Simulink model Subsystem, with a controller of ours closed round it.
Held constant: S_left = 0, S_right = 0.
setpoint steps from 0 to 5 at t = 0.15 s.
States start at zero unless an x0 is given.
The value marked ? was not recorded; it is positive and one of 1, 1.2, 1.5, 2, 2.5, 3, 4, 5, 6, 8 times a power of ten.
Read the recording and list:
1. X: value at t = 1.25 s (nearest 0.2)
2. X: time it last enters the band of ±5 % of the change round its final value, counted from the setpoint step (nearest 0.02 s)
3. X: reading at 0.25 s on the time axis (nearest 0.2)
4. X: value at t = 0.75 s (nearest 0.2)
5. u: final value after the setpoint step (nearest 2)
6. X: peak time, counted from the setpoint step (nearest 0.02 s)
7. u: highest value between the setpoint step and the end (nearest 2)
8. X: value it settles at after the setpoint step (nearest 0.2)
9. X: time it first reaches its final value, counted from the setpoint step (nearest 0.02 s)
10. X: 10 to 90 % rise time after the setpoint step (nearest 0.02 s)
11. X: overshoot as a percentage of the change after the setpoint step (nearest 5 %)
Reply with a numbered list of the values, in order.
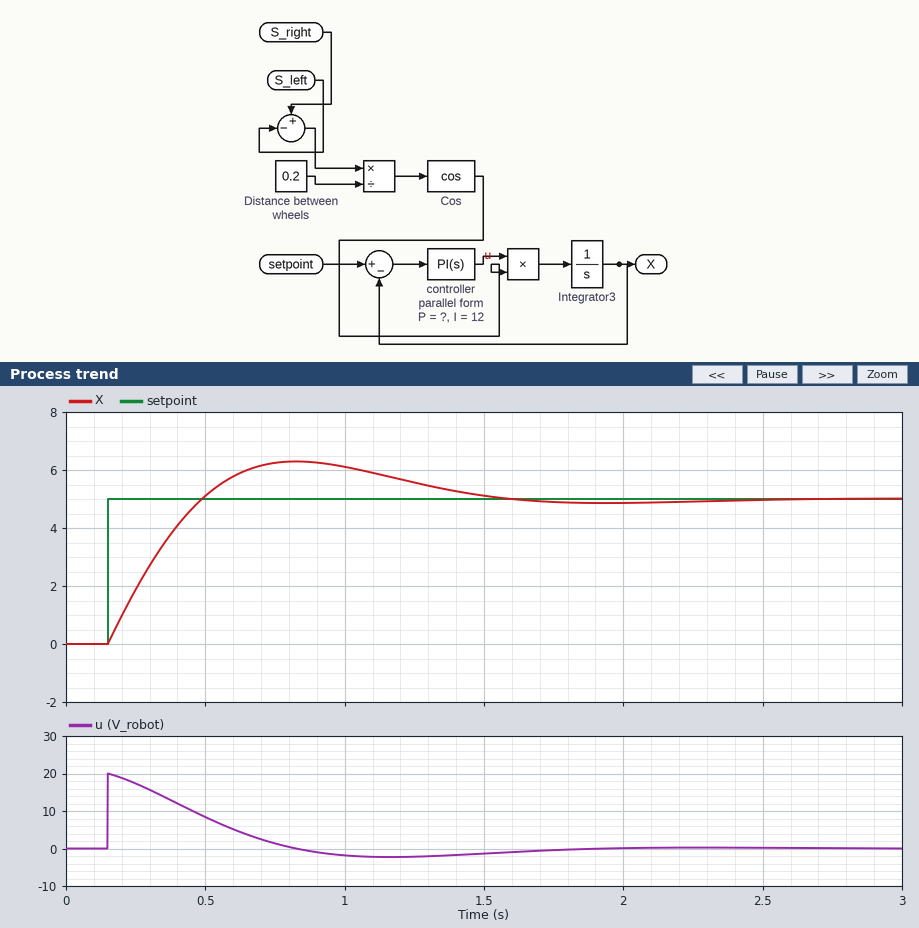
1. 5.6
2. 1.26 s
3. 1.8
4. 6.2
5. 0
6. 0.68 s
7. 20
8. 5.0
9. 0.34 s
10. 0.26 s
11. 25 %
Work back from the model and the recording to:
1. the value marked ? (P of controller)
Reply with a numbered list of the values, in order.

1. 4
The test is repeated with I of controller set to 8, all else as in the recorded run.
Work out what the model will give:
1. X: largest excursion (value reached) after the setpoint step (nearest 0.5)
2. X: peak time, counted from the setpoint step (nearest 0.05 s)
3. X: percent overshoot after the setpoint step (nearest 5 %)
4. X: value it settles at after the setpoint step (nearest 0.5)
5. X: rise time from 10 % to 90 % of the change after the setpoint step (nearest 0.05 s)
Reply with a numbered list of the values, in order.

1. 6.0
2. 0.80 s
3. 20 %
4. 5.0
5. 0.30 s
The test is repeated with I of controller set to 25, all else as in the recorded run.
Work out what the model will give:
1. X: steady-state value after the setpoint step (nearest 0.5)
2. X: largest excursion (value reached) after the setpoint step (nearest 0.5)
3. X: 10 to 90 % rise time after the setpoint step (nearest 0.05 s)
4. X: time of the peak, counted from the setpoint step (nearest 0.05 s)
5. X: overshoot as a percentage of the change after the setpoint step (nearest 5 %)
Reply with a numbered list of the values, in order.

1. 5.0
2. 7.0
3. 0.20 s
4. 0.50 s
5. 35 %
